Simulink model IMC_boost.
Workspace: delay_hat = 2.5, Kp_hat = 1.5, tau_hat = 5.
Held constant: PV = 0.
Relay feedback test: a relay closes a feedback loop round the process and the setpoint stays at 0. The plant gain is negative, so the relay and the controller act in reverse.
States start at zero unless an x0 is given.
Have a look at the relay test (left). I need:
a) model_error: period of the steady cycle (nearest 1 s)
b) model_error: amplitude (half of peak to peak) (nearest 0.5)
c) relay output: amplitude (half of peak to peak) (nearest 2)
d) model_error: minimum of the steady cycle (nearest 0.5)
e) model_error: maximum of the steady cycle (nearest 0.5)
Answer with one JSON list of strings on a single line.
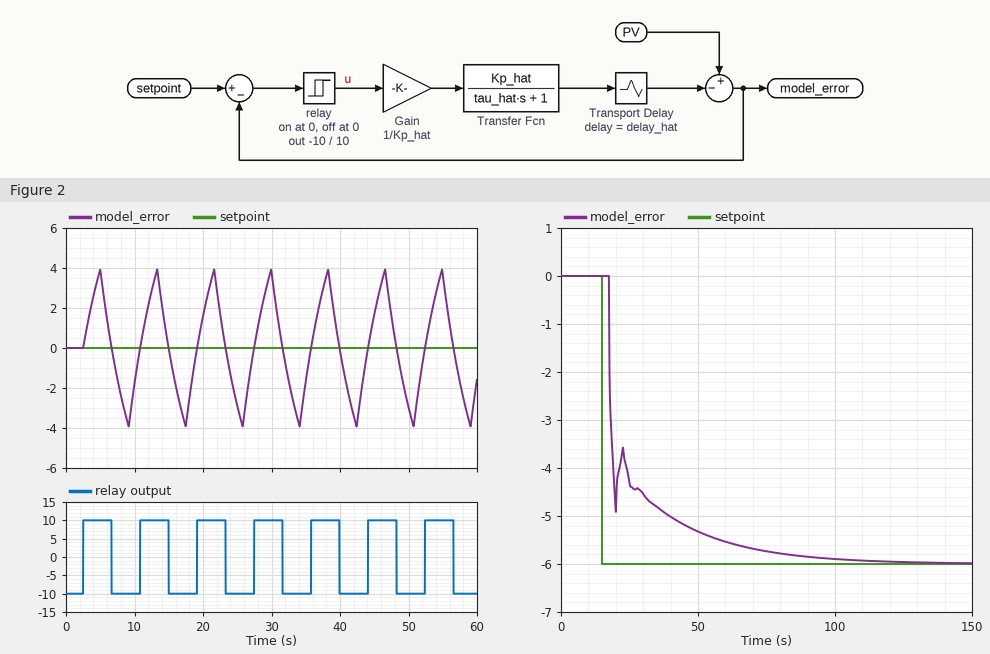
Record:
["8 s", "4.0", "10", "-4.0", "4.0"]
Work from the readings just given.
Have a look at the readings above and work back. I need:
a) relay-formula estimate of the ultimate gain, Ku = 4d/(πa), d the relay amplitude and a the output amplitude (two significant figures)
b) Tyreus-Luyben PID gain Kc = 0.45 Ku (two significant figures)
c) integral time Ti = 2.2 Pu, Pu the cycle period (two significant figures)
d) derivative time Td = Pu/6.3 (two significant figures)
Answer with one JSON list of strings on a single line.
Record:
["3.2", "1.4", "18 s", "1.3 s"]
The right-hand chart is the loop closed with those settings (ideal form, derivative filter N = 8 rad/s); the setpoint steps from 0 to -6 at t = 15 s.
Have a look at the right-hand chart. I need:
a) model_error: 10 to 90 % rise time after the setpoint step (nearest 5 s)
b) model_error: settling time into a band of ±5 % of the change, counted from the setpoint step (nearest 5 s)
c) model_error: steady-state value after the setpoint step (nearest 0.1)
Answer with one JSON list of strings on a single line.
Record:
["35 s", "55 s", "-6.0"]
